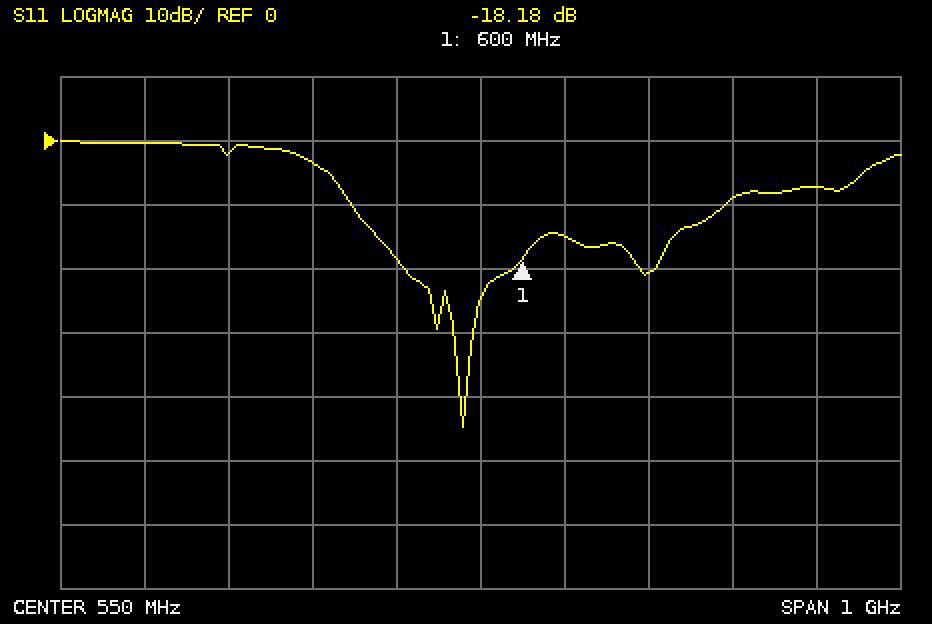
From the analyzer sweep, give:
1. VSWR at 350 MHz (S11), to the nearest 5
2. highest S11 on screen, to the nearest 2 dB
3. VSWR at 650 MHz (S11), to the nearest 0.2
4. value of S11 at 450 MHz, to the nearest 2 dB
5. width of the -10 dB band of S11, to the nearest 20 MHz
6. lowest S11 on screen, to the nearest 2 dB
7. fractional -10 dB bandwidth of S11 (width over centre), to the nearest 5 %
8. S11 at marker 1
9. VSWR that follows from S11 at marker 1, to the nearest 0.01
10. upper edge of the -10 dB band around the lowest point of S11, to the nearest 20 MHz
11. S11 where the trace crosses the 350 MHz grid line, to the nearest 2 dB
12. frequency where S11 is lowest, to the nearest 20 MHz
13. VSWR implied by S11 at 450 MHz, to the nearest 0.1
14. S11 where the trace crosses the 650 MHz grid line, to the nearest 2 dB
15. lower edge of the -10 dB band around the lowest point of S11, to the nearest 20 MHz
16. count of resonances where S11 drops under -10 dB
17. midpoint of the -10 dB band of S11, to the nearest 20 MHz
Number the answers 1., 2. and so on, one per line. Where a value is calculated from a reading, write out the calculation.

1. |Γ| = 10^(-4/20) = 0.6310; VSWR = (1 + 0.6310)/(1 − 0.6310) ≈ 4.42, so 5 to the nearest 5
2. 0 dB
3. |Γ| = 10^(-14/20) = 0.1995; VSWR = (1 + 0.1995)/(1 − 0.1995) ≈ 1.50, so 1.4 to the nearest 0.2
4. -18 dB
5. 840 MHz − 400 MHz = 440 MHz
6. -44 dB
7. 440 MHz / 620 MHz ≈ 71.0 %, so 70 % to the nearest 5 %
8. -18.18 dB
9. (1 + 0.1233)/(1 − 0.1233) ≈ 1.28
10. 840 MHz
11. -4 dB
12. 520 MHz
13. |Γ| = 10^(-18/20) = 0.1259; VSWR = (1 + 0.1259)/(1 − 0.1259) ≈ 1.3
14. -14 dB
15. 400 MHz
16. 3
17. 620 MHz
